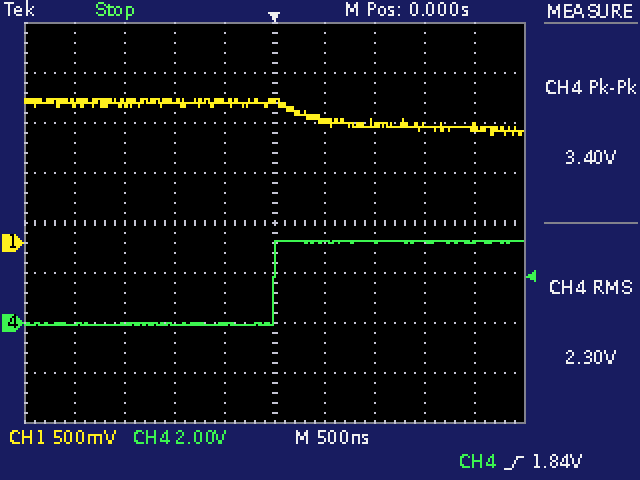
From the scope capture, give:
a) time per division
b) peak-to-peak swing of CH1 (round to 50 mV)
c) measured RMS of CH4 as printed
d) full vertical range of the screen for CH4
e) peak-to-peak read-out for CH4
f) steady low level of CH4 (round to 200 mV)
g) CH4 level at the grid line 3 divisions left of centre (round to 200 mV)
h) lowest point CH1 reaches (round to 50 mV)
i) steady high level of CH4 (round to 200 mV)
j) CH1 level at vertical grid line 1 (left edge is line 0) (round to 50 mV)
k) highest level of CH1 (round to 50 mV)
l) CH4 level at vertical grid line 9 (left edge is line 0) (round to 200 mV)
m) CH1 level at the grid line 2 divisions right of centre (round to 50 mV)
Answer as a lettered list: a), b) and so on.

a) 500 ns
b) 350 mV
c) 2.30 V
d) 16 V
e) 3.40 V
f) 0.0 V
g) 0.0 V
h) 1.10 V
i) 3.2 V
j) 1.40 V
k) 1.45 V
l) 3.2 V
m) 1.20 V
